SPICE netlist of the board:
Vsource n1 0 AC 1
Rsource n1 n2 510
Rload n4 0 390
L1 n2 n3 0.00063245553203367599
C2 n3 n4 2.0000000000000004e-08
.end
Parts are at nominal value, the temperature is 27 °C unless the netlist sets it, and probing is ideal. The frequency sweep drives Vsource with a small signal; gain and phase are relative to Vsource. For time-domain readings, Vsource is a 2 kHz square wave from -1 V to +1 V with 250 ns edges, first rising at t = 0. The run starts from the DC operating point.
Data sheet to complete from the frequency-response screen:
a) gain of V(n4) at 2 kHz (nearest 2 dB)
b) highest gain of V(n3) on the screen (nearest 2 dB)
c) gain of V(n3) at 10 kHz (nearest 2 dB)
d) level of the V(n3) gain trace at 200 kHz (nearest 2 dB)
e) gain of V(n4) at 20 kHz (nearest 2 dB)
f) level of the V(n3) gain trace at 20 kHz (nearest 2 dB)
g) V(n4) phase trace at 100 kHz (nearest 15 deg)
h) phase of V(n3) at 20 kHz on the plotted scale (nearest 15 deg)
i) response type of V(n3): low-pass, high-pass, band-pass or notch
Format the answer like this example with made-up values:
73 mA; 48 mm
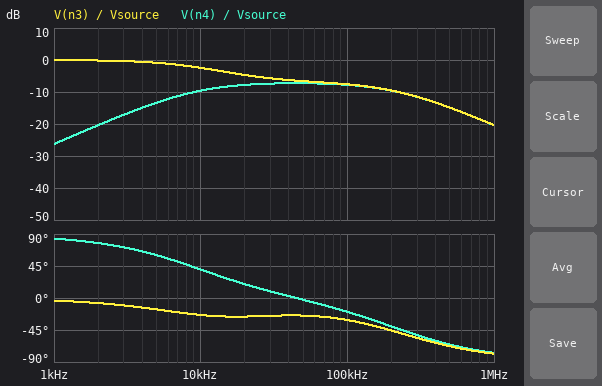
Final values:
-20 dB; 0 dB; -2 dB; -10 dB; -8 dB; -4 dB; -15 deg; -30 deg; low-pass
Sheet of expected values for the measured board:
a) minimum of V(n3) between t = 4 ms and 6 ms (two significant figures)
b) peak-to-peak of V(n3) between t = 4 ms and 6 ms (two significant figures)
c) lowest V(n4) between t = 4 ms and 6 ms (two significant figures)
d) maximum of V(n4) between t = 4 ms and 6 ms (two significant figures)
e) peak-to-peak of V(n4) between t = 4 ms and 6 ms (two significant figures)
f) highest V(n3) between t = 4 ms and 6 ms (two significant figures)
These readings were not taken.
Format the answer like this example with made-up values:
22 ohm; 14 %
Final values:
-1.0 V; 2.0 V; -790 mV; 790 mV; 1.6 V; 1.0 V
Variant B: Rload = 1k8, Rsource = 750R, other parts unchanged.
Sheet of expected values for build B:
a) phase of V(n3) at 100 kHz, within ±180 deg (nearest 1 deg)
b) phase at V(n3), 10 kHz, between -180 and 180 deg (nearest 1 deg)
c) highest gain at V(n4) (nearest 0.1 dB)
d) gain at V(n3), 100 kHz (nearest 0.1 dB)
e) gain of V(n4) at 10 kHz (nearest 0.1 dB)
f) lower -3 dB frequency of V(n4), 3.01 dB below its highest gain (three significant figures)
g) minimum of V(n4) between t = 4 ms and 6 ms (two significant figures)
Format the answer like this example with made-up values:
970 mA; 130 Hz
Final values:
-10 deg; -7 deg; -3.0 dB; -3.1 dB; -3.4 dB; 3.11 kHz; -1.4 V
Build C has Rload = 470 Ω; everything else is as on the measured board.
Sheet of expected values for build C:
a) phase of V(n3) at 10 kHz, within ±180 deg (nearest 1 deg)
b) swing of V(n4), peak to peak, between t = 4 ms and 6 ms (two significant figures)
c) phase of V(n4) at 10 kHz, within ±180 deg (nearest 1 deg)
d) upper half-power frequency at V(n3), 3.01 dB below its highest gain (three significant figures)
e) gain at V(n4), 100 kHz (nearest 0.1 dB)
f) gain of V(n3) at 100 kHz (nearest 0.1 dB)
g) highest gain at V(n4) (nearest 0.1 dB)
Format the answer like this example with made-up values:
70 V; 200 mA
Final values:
-22 deg; 1.8 V; 38 deg; 11.8 kHz; -6.8 dB; -6.7 dB; -6.4 dB
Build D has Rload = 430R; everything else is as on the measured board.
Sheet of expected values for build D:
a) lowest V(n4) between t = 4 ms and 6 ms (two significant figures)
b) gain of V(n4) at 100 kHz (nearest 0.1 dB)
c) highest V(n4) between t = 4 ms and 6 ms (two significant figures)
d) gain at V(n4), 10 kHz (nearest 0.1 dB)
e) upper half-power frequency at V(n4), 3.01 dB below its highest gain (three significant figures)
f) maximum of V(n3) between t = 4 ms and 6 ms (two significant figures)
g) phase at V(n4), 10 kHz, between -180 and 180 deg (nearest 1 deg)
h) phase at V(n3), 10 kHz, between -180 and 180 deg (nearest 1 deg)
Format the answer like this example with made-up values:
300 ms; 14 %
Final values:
-840 mV; -7.3 dB; 840 mV; -9.0 dB; 245 kHz; 1.0 V; 39 deg; -23 deg
